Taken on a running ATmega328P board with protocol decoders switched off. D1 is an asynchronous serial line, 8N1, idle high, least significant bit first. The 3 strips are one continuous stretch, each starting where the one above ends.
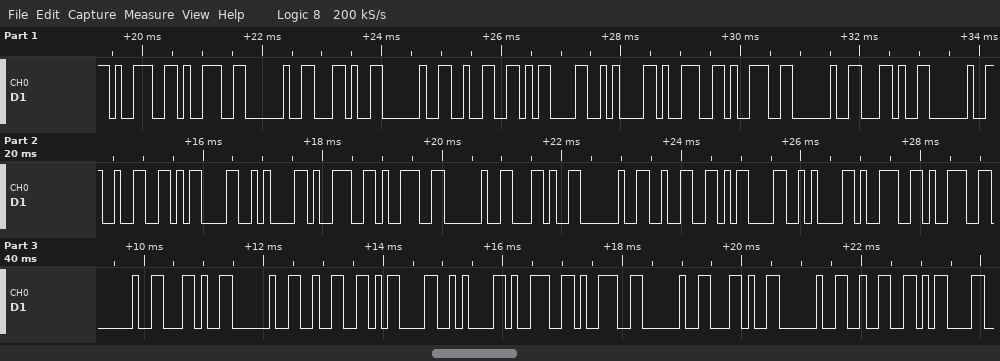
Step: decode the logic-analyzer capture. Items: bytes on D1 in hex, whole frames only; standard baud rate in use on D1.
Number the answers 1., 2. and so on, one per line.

1. 39 39 20 2C 20 32 0D 0A 39 39 20 2C 20 32 0D 0A 39 39 20 2C 20 32 0D 0A 39 39 20 2C 20 32 0D 0A 39 39 20 2C 20 32 0D
2. 9600 baud
